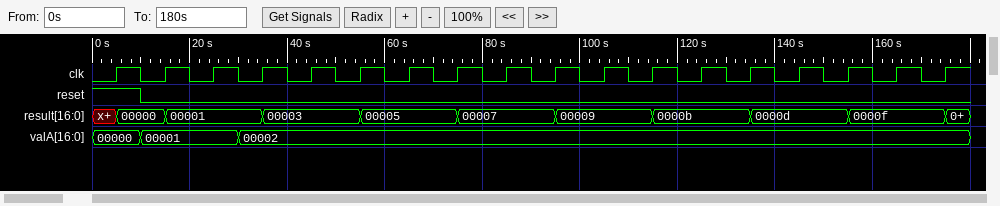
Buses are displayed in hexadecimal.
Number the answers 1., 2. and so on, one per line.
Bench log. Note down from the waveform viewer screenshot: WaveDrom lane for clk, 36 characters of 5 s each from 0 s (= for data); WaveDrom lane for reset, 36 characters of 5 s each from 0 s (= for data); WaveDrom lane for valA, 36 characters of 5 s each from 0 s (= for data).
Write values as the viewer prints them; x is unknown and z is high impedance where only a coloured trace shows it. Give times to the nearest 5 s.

1. {name: 'clk', wave: '010101010101010101010101010101010101'}
2. {name: 'reset', wave: '1.0.................................'}
3. {name: 'valA', wave: '=.=...=.............................', data: '00000 00001 00002'}
